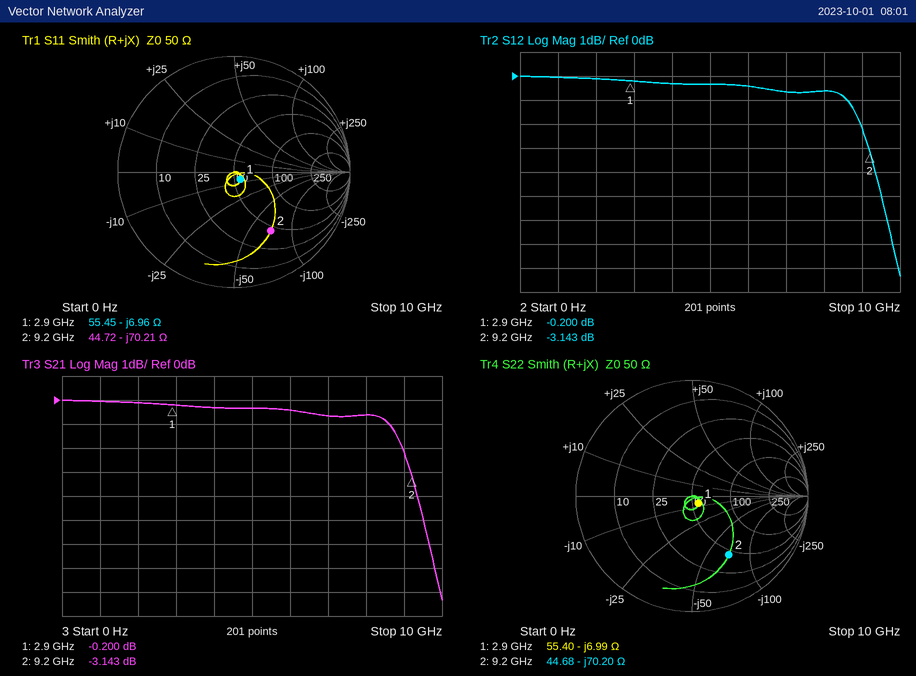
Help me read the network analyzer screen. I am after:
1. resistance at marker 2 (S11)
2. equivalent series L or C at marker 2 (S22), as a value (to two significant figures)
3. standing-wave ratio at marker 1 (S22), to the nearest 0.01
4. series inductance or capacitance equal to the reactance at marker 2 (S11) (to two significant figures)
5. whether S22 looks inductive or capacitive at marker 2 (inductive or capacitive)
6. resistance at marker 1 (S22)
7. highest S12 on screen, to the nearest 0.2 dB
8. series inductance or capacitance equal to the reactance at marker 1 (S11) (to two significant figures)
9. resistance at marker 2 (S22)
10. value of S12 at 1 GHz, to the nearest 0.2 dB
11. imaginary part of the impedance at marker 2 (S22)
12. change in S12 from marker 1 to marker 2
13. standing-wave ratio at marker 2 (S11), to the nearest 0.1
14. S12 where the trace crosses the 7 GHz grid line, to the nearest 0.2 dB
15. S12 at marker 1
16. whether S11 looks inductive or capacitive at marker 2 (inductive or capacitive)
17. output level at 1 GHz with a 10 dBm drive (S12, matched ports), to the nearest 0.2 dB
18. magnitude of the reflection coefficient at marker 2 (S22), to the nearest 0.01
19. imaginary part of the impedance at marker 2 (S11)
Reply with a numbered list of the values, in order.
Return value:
1. 44.72 Ω
2. 250 fF
3. 1.18
4. 250 fF
5. capacitive
6. 55.40 Ω
7. 0.0 dB
8. 7.9 pF
9. 44.68 Ω
10. 0.0 dB
11. -70.20 Ω
12. -2.943 dB
13. 4.0
14. -0.6 dB
15. -0.200 dB
16. capacitive
17. 10.0 dBm
18. 0.60
19. -70.21 Ω
